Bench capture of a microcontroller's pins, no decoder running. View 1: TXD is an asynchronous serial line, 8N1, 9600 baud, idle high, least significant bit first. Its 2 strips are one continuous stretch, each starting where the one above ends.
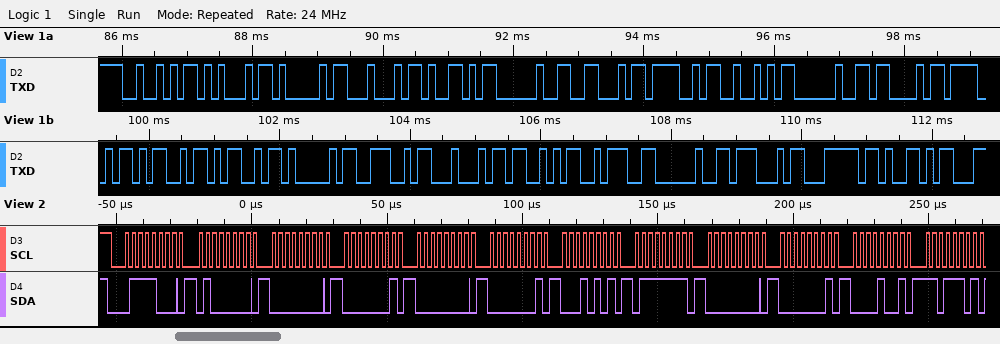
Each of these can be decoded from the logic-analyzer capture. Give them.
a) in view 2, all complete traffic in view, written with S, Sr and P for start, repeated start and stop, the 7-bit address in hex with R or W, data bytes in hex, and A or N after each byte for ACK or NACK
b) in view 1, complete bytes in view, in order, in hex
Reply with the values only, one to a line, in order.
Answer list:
S 3CW A 40 A 00 A 01 A 00 A 01 A 15 A 7F A 00 A 01 A 09 A DD A
0x52 0x45 0x41 0x44 0x59 0x20 0x46 0x4F 0x52 0x20 0x43 0x4F 0x4D 0x4D 0x41 0x4E 0x44 0x53 0x3A 0x20 0x47 0x7C 0x59
